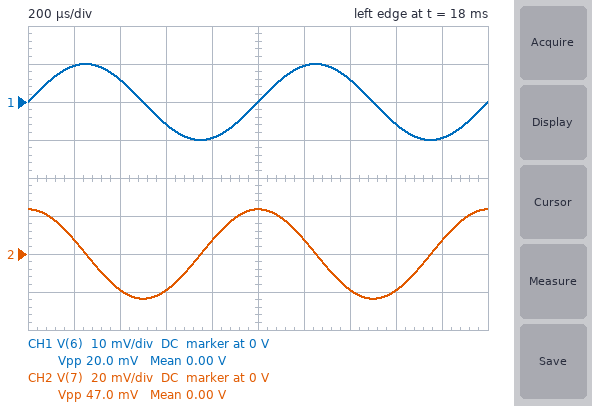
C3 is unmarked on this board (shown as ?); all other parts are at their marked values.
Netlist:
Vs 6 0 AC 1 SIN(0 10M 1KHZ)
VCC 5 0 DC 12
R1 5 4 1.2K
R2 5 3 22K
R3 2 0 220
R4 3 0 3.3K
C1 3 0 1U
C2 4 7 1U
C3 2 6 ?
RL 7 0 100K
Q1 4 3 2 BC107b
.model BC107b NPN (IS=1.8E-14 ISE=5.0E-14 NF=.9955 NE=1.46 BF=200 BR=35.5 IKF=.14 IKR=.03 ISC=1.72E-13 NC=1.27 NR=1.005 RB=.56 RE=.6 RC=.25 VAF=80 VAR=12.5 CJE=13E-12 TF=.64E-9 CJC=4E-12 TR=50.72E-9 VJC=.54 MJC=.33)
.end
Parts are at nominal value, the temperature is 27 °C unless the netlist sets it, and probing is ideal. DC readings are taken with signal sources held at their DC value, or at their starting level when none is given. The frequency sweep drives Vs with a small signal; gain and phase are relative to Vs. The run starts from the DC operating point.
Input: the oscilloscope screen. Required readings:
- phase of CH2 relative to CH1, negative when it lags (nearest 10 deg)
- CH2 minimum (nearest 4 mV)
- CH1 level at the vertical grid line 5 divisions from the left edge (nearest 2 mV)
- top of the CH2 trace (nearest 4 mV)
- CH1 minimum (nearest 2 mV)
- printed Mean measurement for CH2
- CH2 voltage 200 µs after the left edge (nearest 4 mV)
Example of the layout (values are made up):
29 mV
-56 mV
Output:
90 deg
-24 mV
0 V
24 mV
-10 mV
0.00 V
8 mV
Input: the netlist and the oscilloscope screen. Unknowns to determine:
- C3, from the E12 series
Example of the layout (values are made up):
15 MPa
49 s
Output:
330 nF
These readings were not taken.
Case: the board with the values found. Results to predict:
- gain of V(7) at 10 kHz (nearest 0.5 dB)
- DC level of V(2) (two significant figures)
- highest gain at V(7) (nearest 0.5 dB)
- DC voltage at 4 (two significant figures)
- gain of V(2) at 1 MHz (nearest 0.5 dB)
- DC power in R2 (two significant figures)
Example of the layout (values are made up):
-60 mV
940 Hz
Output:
27.5 dB
830 mV
43.5 dB
7.5 V
0 dB
5.0 mW
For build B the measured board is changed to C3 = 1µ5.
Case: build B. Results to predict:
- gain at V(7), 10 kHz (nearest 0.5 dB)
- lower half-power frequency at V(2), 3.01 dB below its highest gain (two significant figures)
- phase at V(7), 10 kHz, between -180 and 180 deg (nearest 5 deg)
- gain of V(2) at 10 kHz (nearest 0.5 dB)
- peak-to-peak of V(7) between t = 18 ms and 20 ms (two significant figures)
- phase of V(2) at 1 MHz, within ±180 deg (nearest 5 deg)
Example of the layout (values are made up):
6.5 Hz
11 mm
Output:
38.5 dB
14 kHz
55 deg
-4.5 dB
210 mV
0 deg
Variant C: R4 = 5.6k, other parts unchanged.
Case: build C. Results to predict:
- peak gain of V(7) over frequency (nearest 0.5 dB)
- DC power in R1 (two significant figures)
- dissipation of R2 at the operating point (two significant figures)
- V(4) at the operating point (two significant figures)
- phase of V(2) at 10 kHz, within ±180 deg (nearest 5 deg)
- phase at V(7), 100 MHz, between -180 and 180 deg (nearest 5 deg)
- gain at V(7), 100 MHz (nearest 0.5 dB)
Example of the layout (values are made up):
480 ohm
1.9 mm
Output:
47.5 dB
59 mW
4.3 mW
3.6 V
85 deg
-70 deg
40.5 dB
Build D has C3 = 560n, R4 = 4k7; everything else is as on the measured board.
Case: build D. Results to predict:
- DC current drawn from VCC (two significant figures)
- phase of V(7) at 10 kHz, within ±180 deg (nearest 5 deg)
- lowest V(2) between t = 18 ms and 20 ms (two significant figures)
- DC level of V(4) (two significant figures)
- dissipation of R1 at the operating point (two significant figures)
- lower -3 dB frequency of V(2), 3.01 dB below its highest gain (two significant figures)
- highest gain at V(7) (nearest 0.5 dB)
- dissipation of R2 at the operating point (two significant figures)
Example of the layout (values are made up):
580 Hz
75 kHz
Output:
6.3 mA
80 deg
1.3 V
5.0 V
41 mW
52 kHz
46.5 dB
4.6 mW
